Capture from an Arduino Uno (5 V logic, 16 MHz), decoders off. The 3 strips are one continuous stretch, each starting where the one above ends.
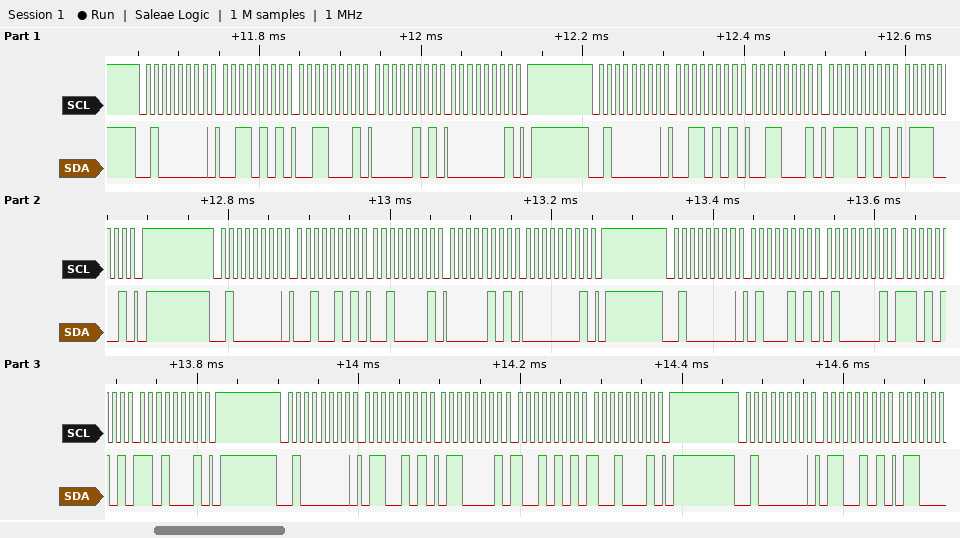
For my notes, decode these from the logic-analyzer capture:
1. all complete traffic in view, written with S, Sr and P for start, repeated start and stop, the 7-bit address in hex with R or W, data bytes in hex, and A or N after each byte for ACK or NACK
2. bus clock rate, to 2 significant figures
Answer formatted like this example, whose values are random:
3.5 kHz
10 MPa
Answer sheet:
S 20W A 35 A 31 A 05 A 01 A P S 20W A 35 A 31 A 75 A 71 A P S 20W A 25 A 21 A 05 A 01 A P S 20W A 45 A 41 A D5 A D1 A P S 20W A 65 A 61 A 95 A 91 A P S 20W A 65 A
100 kHz
